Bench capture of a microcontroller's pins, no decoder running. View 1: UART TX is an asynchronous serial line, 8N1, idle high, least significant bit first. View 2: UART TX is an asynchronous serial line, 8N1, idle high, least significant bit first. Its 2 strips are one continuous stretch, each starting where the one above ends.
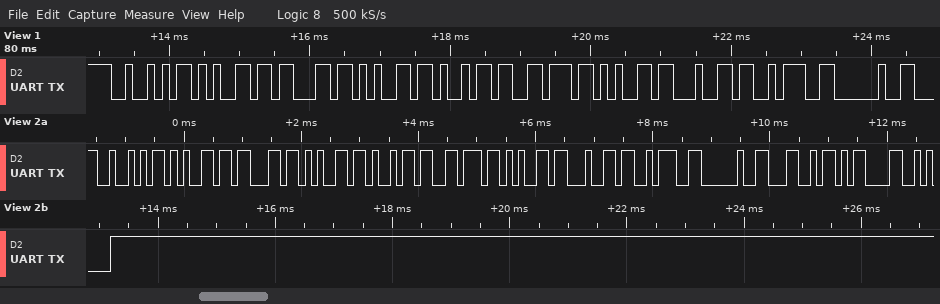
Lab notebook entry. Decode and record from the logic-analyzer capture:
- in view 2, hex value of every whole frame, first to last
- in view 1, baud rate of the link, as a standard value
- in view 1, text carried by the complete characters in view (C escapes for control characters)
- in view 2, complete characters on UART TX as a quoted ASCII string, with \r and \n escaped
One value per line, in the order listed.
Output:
52 65 63 65 69 76 65 64 3A 20 4C 0D 0A
9600 baud
"Received: "
"Received: L\r\n"
